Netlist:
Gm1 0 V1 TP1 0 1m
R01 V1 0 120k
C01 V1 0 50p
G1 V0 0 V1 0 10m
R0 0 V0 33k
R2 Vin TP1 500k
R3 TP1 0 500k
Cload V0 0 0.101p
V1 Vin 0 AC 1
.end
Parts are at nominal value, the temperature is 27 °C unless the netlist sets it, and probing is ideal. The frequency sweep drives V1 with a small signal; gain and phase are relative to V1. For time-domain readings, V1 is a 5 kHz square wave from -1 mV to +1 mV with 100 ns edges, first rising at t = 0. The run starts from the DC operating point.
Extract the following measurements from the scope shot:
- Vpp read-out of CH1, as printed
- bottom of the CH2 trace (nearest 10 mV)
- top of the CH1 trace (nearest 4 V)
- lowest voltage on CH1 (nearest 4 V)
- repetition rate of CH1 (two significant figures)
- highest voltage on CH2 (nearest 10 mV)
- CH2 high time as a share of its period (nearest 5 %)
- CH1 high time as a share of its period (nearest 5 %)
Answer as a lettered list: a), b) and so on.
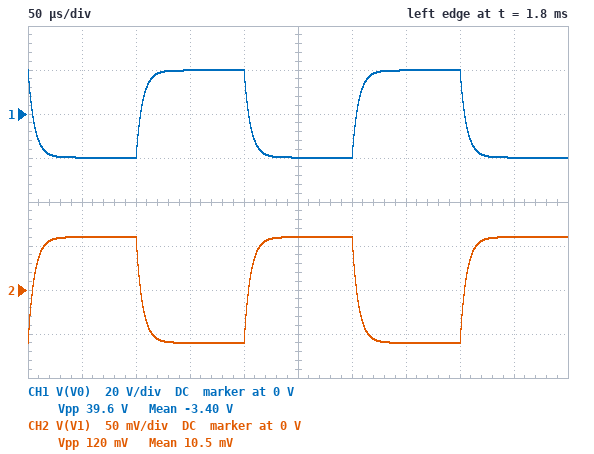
a) 39.6 V
b) -60 mV
c) 20 V
d) -20 V
e) 5.0 kHz
f) 60 mV
g) 50 %
h) 50 %
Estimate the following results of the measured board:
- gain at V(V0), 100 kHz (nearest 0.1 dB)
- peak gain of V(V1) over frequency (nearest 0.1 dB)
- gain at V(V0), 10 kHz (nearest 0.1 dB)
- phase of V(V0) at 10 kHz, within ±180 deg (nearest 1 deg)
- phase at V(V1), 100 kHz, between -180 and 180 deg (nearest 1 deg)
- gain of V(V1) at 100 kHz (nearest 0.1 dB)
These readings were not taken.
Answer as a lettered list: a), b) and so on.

a) 74.1 dB
b) 35.6 dB
c) 85.4 dB
d) 159 deg
e) -75 deg
f) 23.7 dB
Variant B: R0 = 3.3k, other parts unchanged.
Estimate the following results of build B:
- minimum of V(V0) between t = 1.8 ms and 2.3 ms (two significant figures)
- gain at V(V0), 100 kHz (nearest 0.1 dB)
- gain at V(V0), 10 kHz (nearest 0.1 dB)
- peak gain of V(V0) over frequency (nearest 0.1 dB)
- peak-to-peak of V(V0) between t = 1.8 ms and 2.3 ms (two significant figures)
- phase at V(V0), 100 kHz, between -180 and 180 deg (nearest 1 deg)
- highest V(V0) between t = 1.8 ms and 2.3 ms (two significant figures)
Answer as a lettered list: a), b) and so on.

a) -2.0 V
b) 54.1 dB
c) 65.4 dB
d) 65.9 dB
e) 4.0 V
f) 105 deg
g) 2.0 V
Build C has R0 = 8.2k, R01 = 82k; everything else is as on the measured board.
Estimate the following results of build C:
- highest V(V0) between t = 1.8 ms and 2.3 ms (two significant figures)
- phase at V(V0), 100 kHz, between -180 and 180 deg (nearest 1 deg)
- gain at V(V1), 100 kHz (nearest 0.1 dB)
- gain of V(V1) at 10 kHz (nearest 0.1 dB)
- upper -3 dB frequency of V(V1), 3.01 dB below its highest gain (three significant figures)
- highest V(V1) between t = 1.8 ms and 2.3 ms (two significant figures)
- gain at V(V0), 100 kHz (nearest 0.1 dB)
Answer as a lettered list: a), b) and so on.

a) 3.4 V
b) 111 deg
c) 23.4 dB
d) 32.0 dB
e) 38.8 kHz
f) 41 mV
g) 61.7 dB
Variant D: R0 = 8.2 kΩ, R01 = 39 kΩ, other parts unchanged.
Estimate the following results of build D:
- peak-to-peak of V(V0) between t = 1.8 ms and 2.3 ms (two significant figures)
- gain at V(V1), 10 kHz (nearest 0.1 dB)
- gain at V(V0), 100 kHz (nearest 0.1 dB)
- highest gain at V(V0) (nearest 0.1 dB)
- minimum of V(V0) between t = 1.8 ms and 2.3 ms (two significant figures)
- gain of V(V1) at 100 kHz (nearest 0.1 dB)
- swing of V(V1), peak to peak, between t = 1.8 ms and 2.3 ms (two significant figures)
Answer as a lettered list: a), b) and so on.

a) 3.2 V
b) 25.7 dB
c) 60.1 dB
d) 64.1 dB
e) -1.6 V
f) 21.8 dB
g) 39 mV
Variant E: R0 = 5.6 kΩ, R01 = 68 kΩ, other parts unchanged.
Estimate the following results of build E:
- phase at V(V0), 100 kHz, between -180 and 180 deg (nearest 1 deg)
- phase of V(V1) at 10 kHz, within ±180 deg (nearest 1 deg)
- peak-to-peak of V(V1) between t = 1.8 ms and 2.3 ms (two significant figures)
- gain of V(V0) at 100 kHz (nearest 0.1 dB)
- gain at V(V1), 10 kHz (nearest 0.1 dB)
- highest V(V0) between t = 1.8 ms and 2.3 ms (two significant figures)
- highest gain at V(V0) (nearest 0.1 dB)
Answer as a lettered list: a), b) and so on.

a) 115 deg
b) -12 deg
c) 68 mV
d) 58.1 dB
e) 30.4 dB
f) 1.9 V
g) 65.6 dB
